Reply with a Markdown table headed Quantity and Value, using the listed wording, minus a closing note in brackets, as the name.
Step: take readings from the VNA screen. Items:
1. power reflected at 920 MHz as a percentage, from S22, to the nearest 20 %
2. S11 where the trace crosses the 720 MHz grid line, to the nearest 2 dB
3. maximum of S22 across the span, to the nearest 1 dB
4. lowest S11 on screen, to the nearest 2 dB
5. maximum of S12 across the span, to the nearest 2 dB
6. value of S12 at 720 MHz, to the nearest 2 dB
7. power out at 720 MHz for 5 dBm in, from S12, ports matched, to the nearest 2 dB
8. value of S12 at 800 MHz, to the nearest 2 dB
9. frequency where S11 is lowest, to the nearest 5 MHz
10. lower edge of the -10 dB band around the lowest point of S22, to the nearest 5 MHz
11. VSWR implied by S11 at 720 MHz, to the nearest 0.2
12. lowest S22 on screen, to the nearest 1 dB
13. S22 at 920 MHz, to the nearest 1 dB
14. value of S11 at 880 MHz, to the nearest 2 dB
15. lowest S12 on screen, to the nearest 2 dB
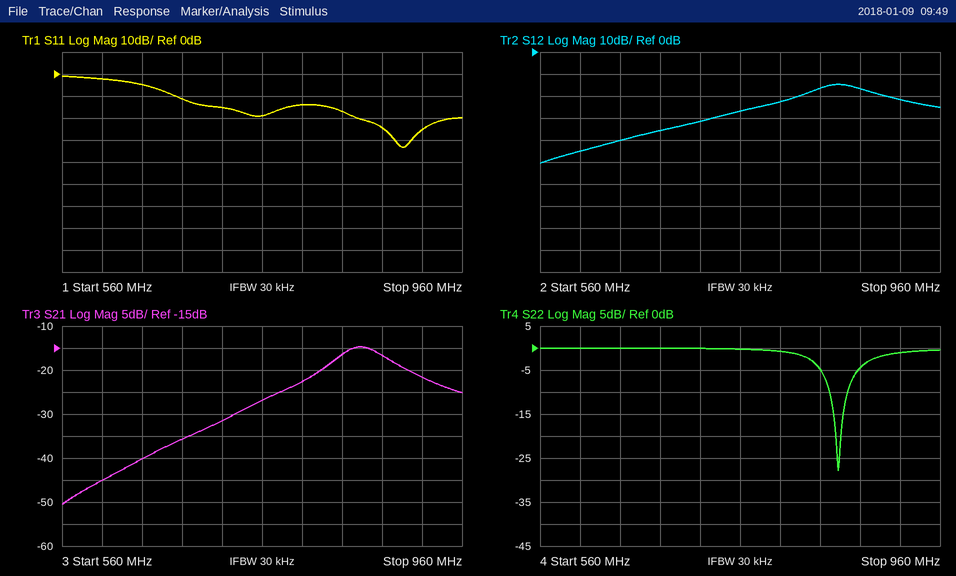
| Quantity | Value |
|---|---|
| power reflected at 920 MHz as a percentage, from S22, to the nearest 20 % | 80 % |
| S11 where the trace crosses the 720 MHz grid line, to the nearest 2 dB | -16 dB |
| maximum of S22 across the span, to the nearest 1 dB | 0 dB |
| lowest S11 on screen, to the nearest 2 dB | -34 dB |
| maximum of S12 across the span, to the nearest 2 dB | -14 dB |
| value of S12 at 720 MHz, to the nearest 2 dB | -32 dB |
| power out at 720 MHz for 5 dBm in, from S12, ports matched, to the nearest 2 dB | -26 dBm |
| value of S12 at 800 MHz, to the nearest 2 dB | -22 dB |
| frequency where S11 is lowest, to the nearest 5 MHz | 900 MHz |
| lower edge of the -10 dB band around the lowest point of S22, to the nearest 5 MHz | 850 MHz |
| VSWR implied by S11 at 720 MHz, to the nearest 0.2 | 1.4 |
| lowest S22 on screen, to the nearest 1 dB | -28 dB |
| S22 at 920 MHz, to the nearest 1 dB | -1 dB |
| value of S11 at 880 MHz, to the nearest 2 dB | -24 dB |
| lowest S12 on screen, to the nearest 2 dB | -50 dB |
